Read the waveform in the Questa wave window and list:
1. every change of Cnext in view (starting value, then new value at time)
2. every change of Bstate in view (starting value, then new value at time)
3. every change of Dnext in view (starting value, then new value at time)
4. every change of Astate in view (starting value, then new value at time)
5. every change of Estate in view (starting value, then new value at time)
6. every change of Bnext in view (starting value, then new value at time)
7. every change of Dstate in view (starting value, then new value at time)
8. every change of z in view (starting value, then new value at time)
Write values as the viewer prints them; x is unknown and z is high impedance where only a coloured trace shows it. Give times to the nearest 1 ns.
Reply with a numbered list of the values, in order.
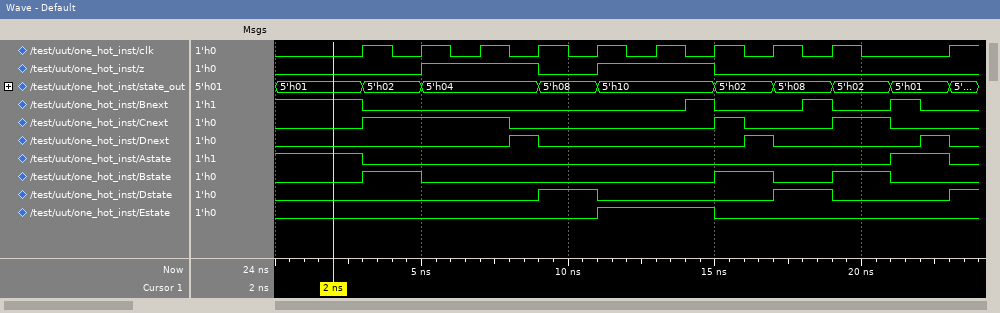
1. 0, 1 at 3 ns, 0 at 8 ns, 1 at 15 ns, 0 at 16 ns, 1 at 19 ns, 0 at 21 ns
2. 0, 1 at 3 ns, 0 at 5 ns, 1 at 15 ns, 0 at 17 ns, 1 at 19 ns, 0 at 21 ns
3. 0, 1 at 8 ns, 0 at 9 ns, 1 at 16 ns, 0 at 17 ns, 1 at 22 ns, 0 at 23 ns
4. 1, 0 at 3 ns, 1 at 21 ns, 0 at 23 ns
5. 0, 1 at 11 ns, 0 at 15 ns
6. 1, 0 at 3 ns, 1 at 14 ns, 0 at 15 ns, 1 at 18 ns, 0 at 19 ns, 1 at 21 ns, 0 at 22 ns
7. 0, 1 at 9 ns, 0 at 11 ns, 1 at 17 ns, 0 at 19 ns, 1 at 23 ns
8. 0, 1 at 5 ns, 0 at 9 ns, 1 at 11 ns, 0 at 15 ns
